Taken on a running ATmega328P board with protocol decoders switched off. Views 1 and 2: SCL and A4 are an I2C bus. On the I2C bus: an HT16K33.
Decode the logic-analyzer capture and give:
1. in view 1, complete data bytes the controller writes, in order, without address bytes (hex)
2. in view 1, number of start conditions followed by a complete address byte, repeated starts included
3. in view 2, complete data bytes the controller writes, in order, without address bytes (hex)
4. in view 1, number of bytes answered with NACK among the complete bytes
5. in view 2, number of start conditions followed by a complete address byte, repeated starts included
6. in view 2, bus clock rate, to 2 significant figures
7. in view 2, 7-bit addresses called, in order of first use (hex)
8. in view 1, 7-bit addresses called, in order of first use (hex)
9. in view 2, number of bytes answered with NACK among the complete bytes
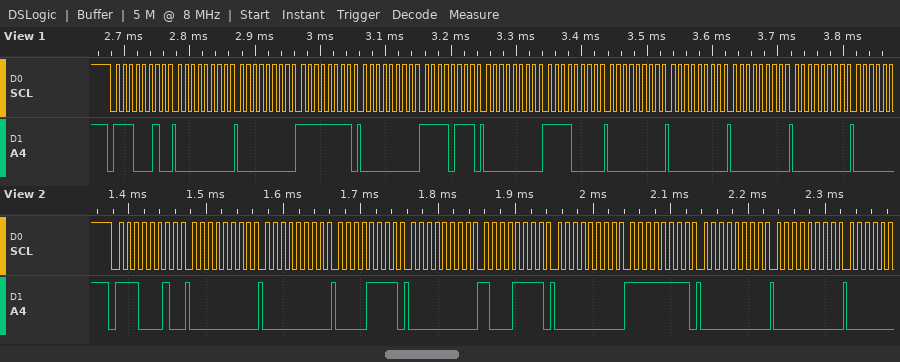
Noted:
00 00 FF 00 F7 00 F0 00 00 00 00
1
00 00 0F 00 8F 00 FF 00 00
0
1
100 kHz
0x71
0x71
0
